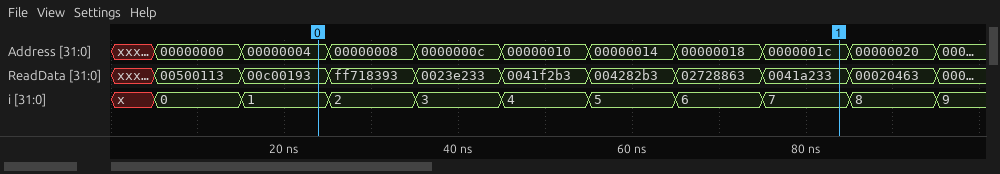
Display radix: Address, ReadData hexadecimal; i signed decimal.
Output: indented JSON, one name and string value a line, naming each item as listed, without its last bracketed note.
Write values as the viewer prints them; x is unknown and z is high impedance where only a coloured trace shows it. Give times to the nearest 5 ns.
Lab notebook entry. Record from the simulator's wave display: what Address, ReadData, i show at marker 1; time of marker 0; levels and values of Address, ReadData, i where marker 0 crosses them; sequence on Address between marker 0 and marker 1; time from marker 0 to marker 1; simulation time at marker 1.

{
  "what Address, ReadData, i show at marker 1": "Address=0000001c, ReadData=0041a233, i=7",
  "time of marker 0": "25 ns",
  "levels and values of Address, ReadData, i where marker 0 crosses them": "Address=00000004, ReadData=00c00193, i=1",
  "sequence on Address between marker 0 and marker 1": "00000004, 00000008, 0000000c, 00000010, 00000014, 00000018, 0000001c",
  "time from marker 0 to marker 1": "60 ns",
  "simulation time at marker 1": "85 ns"
}
